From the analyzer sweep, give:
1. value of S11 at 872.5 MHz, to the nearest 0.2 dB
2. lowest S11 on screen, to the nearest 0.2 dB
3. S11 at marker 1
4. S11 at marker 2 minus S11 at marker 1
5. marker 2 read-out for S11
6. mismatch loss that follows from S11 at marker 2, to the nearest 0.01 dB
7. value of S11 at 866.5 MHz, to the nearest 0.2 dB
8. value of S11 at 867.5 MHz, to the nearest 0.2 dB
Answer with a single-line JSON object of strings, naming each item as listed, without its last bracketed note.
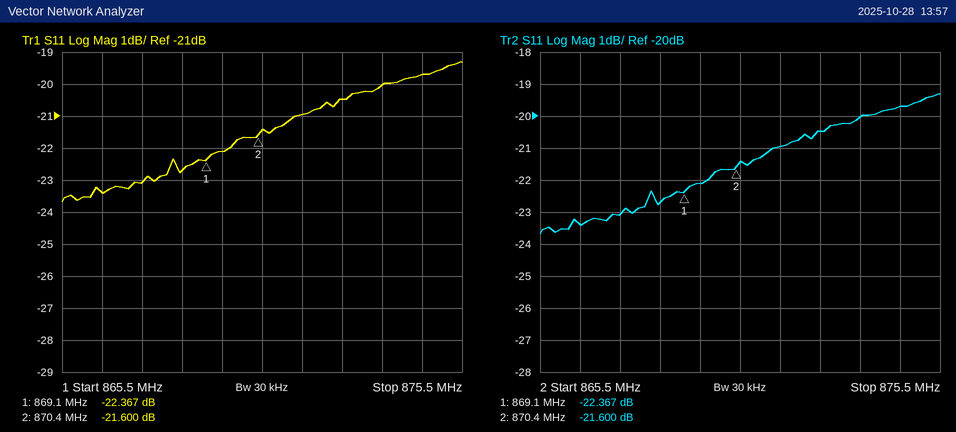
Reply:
{"value of S11 at 872.5 MHz, to the nearest 0.2 dB": "-20.4 dB", "lowest S11 on screen, to the nearest 0.2 dB": "-23.6 dB", "S11 at marker 1": "-22.367 dB", "S11 at marker 2 minus S11 at marker 1": "0.767 dB", "marker 2 read-out for S11": "-21.600 dB", "mismatch loss that follows from S11 at marker 2, to the nearest 0.01 dB": "0.03 dB", "value of S11 at 866.5 MHz, to the nearest 0.2 dB": "-23.4 dB", "value of S11 at 867.5 MHz, to the nearest 0.2 dB": "-23.0 dB"}
